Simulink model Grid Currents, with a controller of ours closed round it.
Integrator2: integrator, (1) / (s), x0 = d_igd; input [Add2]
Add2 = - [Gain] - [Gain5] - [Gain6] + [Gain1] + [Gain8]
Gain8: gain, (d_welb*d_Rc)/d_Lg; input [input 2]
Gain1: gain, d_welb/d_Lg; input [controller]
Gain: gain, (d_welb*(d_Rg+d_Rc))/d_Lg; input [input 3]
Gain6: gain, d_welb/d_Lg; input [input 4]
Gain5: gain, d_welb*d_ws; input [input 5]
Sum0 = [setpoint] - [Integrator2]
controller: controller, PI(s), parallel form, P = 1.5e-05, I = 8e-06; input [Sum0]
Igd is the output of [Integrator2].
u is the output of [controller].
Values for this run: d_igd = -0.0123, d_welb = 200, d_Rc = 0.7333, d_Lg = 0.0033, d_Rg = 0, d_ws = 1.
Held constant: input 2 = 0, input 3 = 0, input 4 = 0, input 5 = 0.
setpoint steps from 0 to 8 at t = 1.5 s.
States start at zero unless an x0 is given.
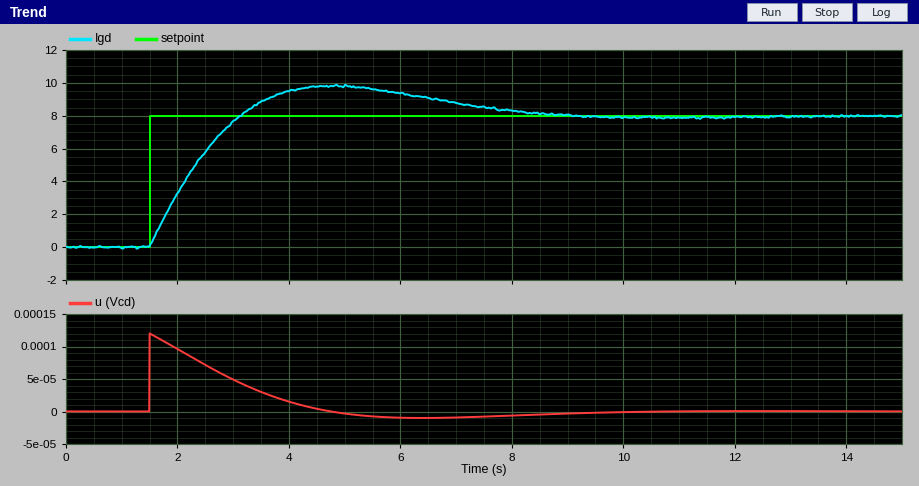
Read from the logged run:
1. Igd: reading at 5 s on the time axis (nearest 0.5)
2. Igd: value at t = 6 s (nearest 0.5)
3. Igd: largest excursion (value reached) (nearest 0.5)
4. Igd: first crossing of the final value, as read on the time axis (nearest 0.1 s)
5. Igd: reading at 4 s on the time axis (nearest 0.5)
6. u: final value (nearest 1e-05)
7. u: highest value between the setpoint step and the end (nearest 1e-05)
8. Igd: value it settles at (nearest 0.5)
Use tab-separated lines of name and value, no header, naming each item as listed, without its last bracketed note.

Igd: reading at 5 s on the time axis	10.0
Igd: value at t = 6 s	9.5
Igd: largest excursion (value reached)	10.0
Igd: first crossing of the final value, as read on the time axis	3.1 s
Igd: reading at 4 s on the time axis	9.5
u: final value	0.00000
u: highest value between the setpoint step and the end	0.00012
Igd: value it settles at	8.0
